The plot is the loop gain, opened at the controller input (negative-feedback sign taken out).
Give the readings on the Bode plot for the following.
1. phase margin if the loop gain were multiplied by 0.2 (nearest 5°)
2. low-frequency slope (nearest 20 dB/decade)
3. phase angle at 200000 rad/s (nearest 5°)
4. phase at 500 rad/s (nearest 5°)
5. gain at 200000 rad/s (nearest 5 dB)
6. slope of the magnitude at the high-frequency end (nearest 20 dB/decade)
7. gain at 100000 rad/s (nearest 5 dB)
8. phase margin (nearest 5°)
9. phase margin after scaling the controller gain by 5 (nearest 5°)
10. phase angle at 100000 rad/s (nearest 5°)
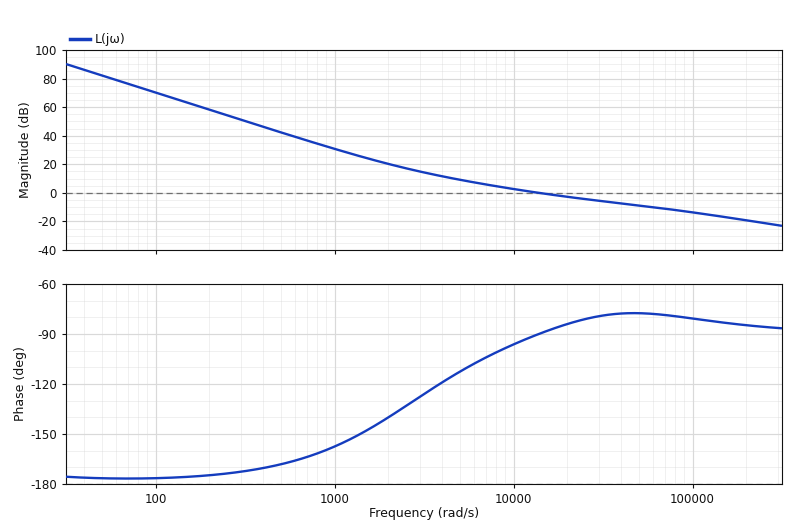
55°
-40 dB/decade
-85°
-170°
-20 dB
-20 dB/decade
-15 dB
90°
100°
-80°
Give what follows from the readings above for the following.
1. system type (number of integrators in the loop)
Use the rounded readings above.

2
